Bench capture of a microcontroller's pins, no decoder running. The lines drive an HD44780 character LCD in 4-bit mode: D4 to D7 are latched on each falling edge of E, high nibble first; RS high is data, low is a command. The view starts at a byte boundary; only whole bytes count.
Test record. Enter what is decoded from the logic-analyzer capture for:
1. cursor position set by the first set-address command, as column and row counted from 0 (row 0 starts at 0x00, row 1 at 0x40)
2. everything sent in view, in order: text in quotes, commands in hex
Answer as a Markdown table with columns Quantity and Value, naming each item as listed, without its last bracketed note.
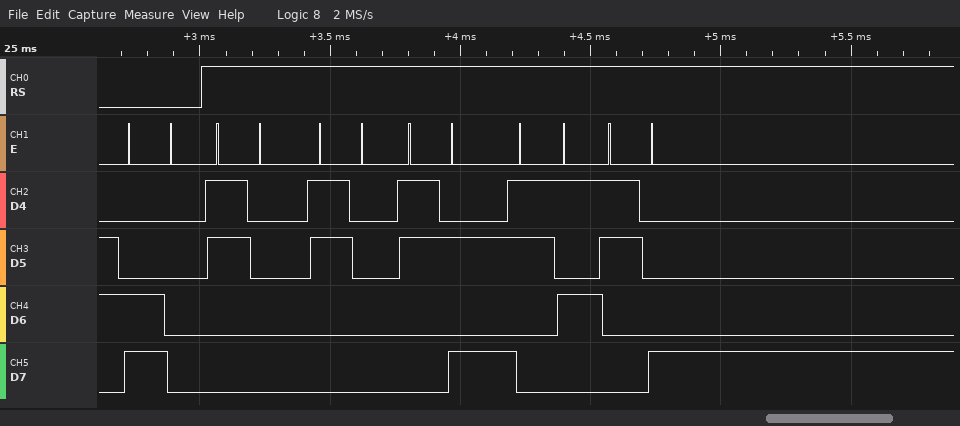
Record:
| Quantity | Value |
|---|---|
| cursor position set by the first set-address command, as column and row counted from 0 | column 0, row 1 |
| everything sent in view, in order: text in quotes, commands in hex | 0xC0 "00:58" |
